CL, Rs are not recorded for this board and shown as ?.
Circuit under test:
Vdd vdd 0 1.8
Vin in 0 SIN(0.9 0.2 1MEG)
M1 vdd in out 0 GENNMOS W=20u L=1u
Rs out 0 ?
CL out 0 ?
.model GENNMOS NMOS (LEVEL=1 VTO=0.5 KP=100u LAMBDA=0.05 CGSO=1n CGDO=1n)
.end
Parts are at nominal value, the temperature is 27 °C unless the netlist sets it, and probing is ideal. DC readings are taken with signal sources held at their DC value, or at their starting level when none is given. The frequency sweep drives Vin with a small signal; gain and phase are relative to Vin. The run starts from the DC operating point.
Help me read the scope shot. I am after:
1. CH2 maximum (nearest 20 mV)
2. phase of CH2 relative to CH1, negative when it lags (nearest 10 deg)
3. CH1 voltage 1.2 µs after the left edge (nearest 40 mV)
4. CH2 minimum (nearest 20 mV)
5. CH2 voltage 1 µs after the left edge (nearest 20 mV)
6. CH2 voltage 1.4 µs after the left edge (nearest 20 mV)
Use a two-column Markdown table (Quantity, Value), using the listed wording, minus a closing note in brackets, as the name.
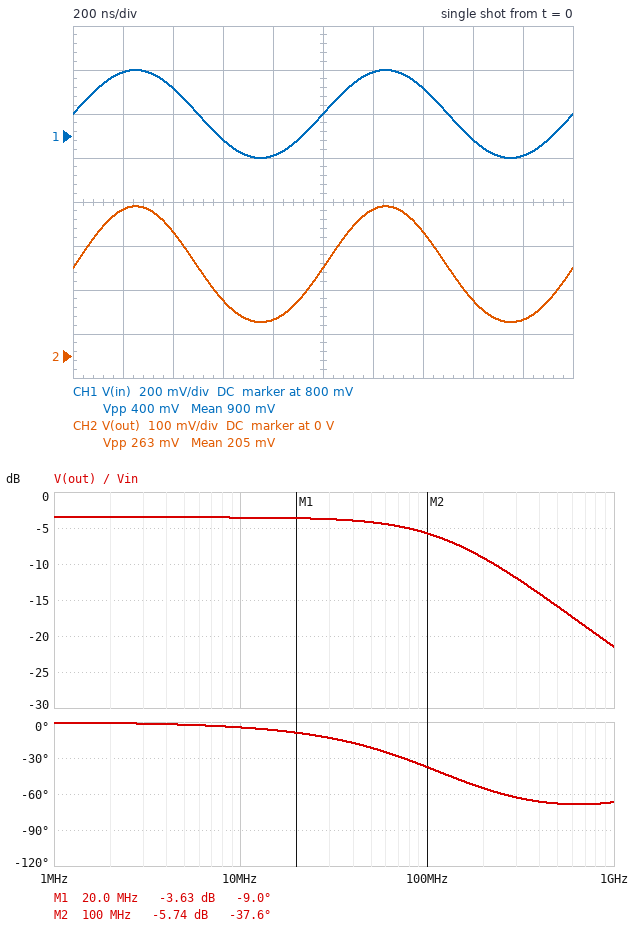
| Quantity | Value |
|---|---|
| CH2 maximum | 340 mV |
| phase of CH2 relative to CH1, negative when it lags | 0 deg |
| CH1 voltage 1.2 µs after the left edge | 1.08 V |
| CH2 minimum | 80 mV |
| CH2 voltage 1 µs after the left edge | 200 mV |
| CH2 voltage 1.4 µs after the left edge | 280 mV |
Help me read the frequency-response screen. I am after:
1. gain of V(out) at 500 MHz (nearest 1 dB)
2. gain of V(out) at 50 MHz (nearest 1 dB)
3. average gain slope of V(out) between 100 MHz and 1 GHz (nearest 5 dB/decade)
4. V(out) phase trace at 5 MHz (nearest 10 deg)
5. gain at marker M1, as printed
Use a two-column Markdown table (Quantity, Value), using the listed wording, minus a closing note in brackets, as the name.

| Quantity | Value |
|---|---|
| gain of V(out) at 500 MHz | -16 dB |
| gain of V(out) at 50 MHz | -4 dB |
| average gain slope of V(out) between 100 MHz and 1 GHz | -15 dB/decade |
| V(out) phase trace at 5 MHz | 0 deg |
| gain at marker M1, as printed | -3.63 dB |
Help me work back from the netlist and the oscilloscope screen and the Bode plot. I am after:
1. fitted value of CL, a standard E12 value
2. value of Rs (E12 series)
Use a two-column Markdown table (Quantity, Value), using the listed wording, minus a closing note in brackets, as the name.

| Quantity | Value |
|---|---|
| fitted value of CL, a standard E12 value | 820 fF |
| value of Rs | 4.7 kΩ |
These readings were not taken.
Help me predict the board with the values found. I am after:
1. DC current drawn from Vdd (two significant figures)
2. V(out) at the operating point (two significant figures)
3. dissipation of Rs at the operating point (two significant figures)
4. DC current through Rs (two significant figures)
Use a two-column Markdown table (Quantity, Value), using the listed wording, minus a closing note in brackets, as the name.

| Quantity | Value |
|---|---|
| DC current drawn from Vdd | 43 µA |
| V(out) at the operating point | 200 mV |
| dissipation of Rs at the operating point | 8.6 µW |
| DC current through Rs | 43 µA |
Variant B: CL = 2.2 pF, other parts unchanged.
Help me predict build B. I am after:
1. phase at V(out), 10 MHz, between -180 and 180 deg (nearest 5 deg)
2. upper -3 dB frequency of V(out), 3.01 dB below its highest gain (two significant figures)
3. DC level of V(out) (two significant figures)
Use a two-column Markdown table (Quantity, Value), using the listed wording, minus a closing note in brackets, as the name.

| Quantity | Value |
|---|---|
| phase at V(out), 10 MHz, between -180 and 180 deg | -10 deg |
| upper -3 dB frequency of V(out), 3.01 dB below its highest gain | 46 MHz |
| DC level of V(out) | 200 mV |
